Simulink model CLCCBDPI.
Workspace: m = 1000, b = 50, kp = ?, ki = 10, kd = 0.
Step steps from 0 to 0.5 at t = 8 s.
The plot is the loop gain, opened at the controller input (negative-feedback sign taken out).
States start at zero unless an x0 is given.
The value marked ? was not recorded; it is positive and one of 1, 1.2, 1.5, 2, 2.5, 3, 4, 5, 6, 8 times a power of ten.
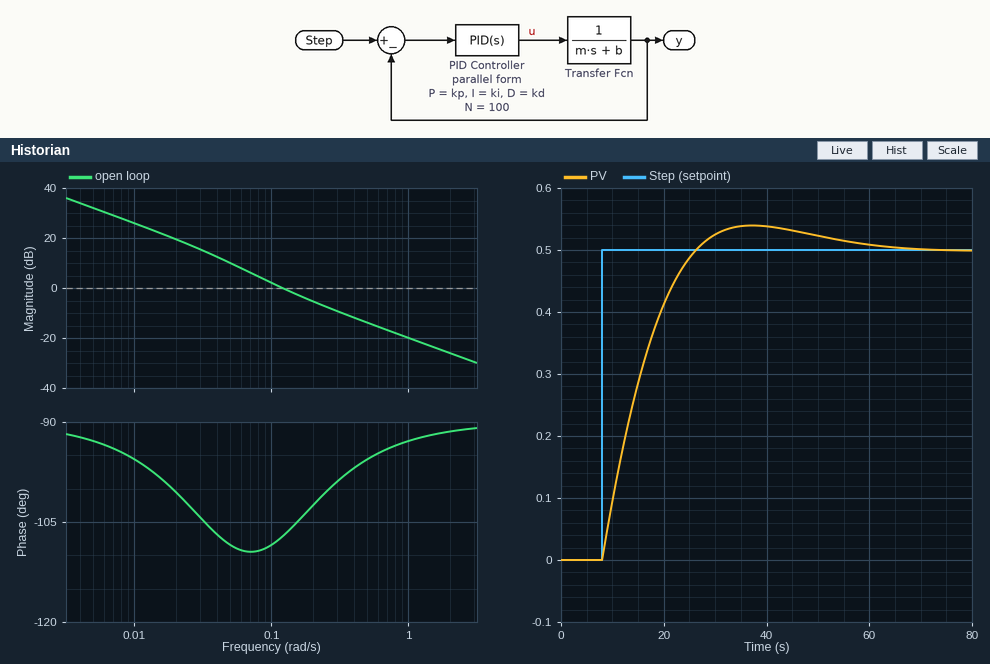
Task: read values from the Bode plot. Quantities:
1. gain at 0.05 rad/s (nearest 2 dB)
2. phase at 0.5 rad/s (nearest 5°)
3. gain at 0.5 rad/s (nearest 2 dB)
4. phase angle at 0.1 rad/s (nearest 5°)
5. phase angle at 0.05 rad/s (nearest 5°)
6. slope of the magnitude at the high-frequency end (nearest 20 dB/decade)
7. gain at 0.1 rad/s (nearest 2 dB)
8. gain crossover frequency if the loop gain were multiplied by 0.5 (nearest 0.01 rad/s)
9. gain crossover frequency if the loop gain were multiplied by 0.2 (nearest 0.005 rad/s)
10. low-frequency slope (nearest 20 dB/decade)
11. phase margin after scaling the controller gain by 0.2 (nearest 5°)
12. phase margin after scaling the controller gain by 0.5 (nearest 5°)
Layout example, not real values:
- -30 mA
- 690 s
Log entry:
- 10 dB
- -95°
- -14 dB
- -110°
- -110°
- -20 dB/decade
- 2 dB
- 0.07 rad/s
- 0.035 rad/s
- -20 dB/decade
- 75°
- 70°
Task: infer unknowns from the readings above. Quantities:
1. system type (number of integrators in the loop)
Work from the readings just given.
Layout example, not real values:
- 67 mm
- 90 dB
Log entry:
- 1
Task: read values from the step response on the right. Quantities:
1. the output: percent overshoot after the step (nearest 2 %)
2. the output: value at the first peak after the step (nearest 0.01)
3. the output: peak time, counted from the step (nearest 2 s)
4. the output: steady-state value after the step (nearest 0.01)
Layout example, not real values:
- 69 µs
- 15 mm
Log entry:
- 8 %
- 0.54
- 30 s
- 0.50
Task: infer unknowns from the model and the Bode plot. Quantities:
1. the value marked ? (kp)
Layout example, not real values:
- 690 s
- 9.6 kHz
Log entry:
- 100
